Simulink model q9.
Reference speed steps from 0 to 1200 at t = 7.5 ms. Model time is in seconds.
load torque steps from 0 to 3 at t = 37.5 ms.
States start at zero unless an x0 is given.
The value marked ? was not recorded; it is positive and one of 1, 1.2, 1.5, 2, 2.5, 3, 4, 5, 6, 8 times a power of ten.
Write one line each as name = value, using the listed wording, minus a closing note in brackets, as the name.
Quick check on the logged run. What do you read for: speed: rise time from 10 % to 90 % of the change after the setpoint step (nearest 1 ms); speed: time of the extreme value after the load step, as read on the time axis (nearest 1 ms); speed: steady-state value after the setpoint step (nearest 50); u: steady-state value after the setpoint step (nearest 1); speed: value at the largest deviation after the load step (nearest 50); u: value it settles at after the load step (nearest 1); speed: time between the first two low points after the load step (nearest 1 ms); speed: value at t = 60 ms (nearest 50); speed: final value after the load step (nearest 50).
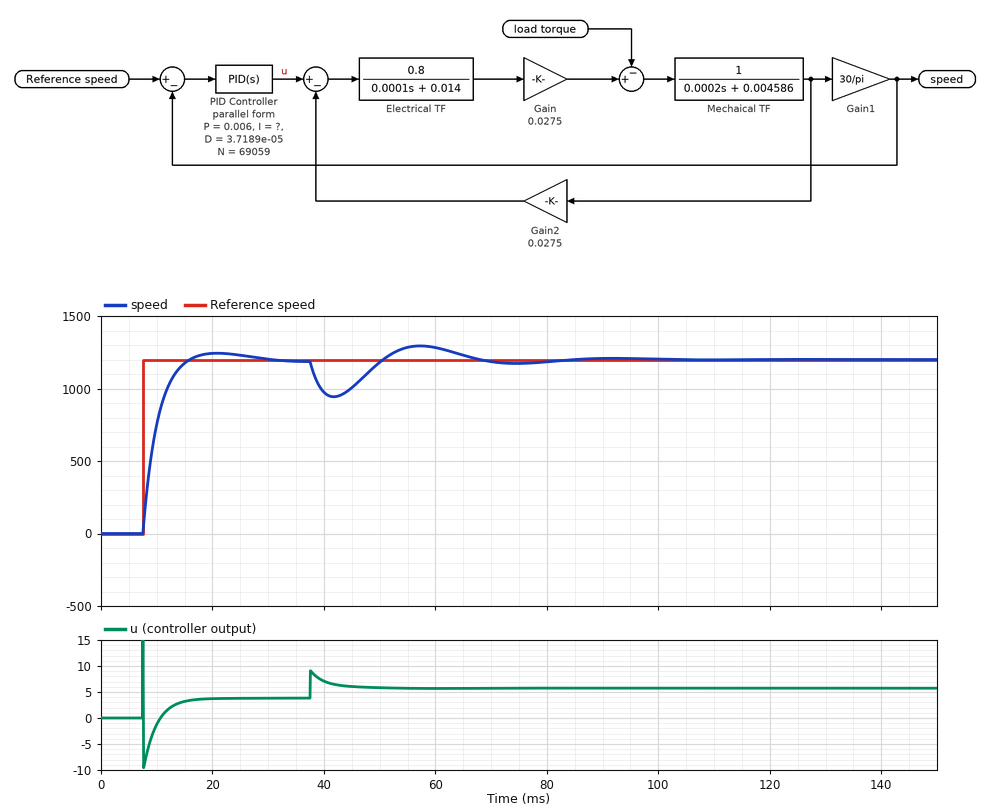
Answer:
speed: rise time from 10 % to 90 % of the change after the setpoint step = 5 ms
speed: time of the extreme value after the load step, as read on the time axis = 42 ms
speed: steady-state value after the setpoint step = 1200
u: steady-state value after the setpoint step = 4
speed: value at the largest deviation after the load step = 950
u: value it settles at after the load step = 6
speed: time between the first two low points after the load step = 33 ms
speed: value at t = 60 ms = 1300
speed: final value after the load step = 1200
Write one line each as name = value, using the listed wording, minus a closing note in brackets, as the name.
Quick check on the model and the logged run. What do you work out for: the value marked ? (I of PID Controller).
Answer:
the value marked ? = 1.5
